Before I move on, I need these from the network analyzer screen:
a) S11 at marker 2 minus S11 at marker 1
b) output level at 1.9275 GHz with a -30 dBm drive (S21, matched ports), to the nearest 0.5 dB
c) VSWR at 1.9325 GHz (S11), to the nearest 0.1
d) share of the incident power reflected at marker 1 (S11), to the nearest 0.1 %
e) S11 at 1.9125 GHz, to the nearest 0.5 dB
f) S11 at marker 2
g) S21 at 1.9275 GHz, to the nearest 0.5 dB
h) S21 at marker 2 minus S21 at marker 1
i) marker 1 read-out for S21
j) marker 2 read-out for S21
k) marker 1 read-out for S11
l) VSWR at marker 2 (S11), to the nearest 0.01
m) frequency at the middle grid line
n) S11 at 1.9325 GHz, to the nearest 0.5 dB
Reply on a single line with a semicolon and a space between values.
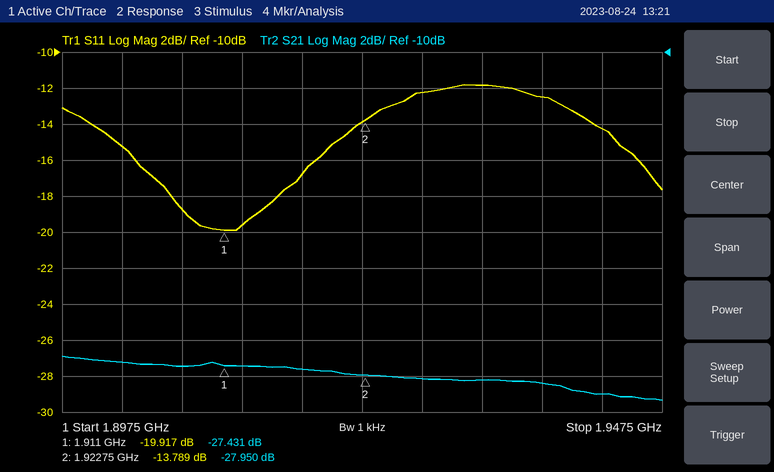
6.128 dB; -58.0 dBm; 1.7; 1.0 %; -19.5 dB; -13.789 dB; -28.0 dB; -0.519 dB; -27.431 dB; -27.950 dB; -19.917 dB; 1.51; 1.9225 GHz; -12.0 dB
